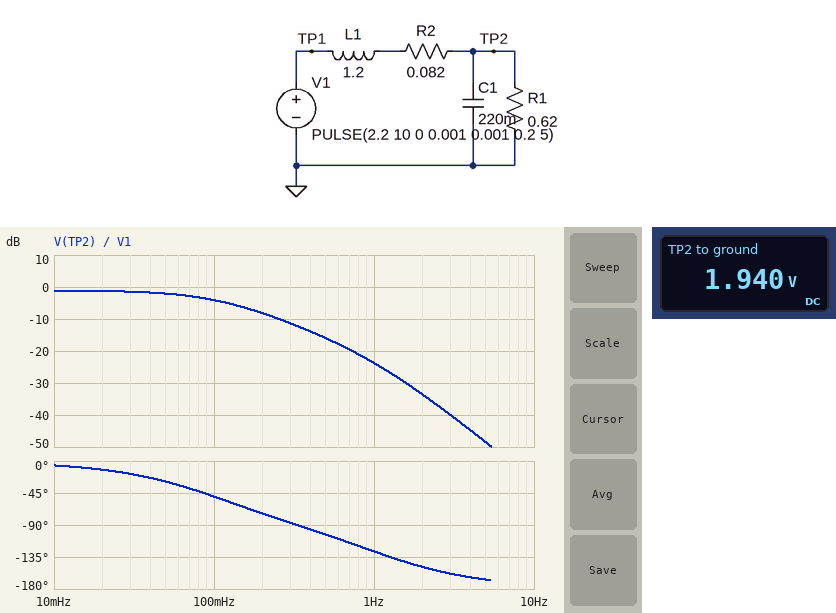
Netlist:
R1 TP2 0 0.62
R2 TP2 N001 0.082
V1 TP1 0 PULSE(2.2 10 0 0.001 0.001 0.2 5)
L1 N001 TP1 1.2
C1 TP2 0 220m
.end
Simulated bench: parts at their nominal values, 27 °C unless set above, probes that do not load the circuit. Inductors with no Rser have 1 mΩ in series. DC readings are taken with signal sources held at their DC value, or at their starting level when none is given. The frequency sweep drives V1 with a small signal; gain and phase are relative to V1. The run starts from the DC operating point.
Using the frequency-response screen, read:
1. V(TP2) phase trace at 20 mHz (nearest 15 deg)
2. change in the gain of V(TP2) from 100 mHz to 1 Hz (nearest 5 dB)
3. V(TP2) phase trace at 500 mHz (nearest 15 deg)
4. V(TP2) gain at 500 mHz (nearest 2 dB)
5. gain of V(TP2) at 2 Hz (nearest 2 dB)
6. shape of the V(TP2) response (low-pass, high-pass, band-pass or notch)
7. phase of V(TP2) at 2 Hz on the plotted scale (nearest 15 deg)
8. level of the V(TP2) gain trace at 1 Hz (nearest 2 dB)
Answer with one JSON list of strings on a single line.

["-15 deg", "-20 dB", "-105 deg", "-16 dB", "-34 dB", "low-pass", "-150 deg", "-24 dB"]
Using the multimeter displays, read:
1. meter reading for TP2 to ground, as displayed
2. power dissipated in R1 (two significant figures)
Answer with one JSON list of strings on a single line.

["1.940 V", "6.1 W"]
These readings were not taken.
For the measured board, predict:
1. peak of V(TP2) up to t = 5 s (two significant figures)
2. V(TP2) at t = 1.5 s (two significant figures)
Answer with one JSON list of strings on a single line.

["2.6 V", "2.3 V"]
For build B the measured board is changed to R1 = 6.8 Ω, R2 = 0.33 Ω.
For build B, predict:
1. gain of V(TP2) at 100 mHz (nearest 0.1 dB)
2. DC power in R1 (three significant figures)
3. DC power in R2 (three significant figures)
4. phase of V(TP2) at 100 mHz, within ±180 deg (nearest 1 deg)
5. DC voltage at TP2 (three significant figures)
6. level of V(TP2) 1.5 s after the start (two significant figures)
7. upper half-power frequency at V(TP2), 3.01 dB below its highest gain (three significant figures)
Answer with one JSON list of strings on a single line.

["0.4 dB", "647 mW", "31.4 mW", "-9 deg", "2.10 V", "2.8 V", "368 mHz"]
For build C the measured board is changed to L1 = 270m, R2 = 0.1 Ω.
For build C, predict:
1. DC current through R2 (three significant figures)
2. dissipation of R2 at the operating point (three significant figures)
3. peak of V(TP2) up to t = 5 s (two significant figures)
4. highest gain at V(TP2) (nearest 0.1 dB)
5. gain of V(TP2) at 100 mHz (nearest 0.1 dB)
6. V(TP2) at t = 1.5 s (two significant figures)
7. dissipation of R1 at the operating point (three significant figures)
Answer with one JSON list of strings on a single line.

["3.05 A", "931 mW", "4.2 V", "-1.3 dB", "-1.4 dB", "1.9 V", "5.77 W"]
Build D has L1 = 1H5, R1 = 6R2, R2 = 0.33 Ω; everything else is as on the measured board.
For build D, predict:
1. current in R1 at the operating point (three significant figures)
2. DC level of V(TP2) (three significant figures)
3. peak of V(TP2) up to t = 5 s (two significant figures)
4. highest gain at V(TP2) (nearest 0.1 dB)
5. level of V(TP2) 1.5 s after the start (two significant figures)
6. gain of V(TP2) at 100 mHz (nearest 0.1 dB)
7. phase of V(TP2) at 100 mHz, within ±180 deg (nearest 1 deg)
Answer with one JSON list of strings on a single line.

["337 mA", "2.09 V", "3.9 V", "5.3 dB", "3.0 V", "0.5 dB", "-12 deg"]
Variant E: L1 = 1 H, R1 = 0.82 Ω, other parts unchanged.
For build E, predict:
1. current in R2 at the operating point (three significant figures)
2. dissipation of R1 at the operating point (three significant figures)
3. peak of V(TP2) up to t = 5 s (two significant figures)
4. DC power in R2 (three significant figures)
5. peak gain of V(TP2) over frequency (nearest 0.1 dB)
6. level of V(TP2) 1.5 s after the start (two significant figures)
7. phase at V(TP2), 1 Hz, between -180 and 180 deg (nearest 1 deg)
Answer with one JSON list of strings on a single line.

["2.44 A", "4.87 W", "3.0 V", "487 mW", "-0.8 dB", "2.4 V", "-134 deg"]
